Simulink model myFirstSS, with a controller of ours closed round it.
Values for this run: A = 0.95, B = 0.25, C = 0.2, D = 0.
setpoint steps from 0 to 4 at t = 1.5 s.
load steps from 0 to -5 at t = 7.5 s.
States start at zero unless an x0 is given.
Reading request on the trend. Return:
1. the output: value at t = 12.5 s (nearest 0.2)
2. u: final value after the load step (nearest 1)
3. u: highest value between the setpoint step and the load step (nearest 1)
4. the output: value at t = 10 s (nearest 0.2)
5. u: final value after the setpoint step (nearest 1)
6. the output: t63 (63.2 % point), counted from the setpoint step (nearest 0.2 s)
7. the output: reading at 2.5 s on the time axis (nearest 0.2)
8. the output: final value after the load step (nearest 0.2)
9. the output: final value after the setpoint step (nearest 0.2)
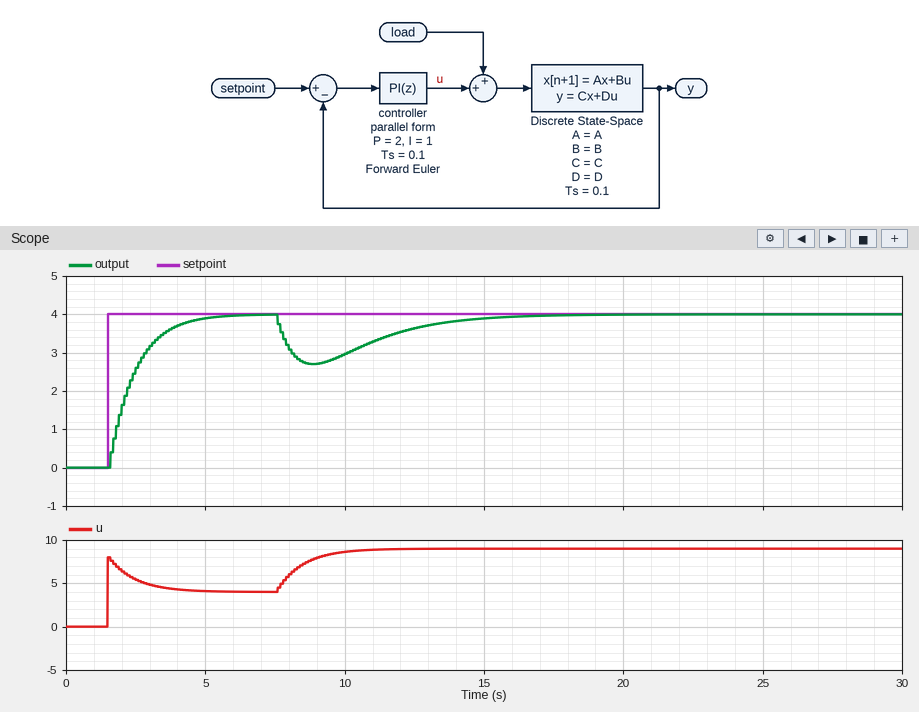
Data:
3.6
9
8
3.0
4
1.0 s
2.6
4.0
4.0
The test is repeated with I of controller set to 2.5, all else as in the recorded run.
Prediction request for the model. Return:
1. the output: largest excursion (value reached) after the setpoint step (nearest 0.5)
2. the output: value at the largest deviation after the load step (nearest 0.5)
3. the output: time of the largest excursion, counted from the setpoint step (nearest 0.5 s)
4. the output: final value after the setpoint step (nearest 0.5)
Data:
4.5
3.0
2.5 s
4.0
